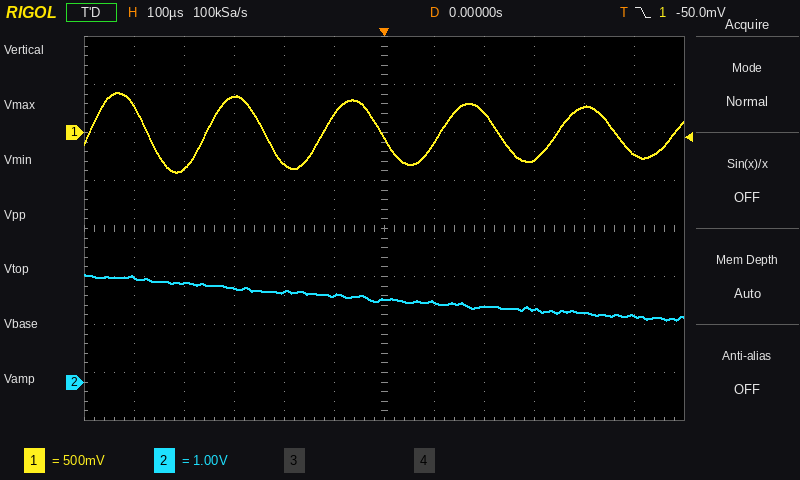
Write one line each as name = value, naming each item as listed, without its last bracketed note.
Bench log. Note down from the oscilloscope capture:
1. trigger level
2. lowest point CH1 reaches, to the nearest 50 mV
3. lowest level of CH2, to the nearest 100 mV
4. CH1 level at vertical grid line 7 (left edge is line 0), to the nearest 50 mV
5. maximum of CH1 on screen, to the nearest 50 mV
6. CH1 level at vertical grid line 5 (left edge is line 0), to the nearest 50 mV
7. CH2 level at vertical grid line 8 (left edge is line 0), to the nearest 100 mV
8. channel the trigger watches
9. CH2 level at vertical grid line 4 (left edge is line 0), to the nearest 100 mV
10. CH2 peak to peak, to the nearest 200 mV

trigger level = -50.0 mV
lowest point CH1 reaches, to the nearest 50 mV = -400 mV
lowest level of CH2, to the nearest 100 mV = 1.3 V
CH1 level at vertical grid line 7 (left edge is line 0), to the nearest 50 mV = -100 mV
maximum of CH1 on screen, to the nearest 50 mV = 400 mV
CH1 level at vertical grid line 5 (left edge is line 0), to the nearest 50 mV = 200 mV
CH2 level at vertical grid line 8 (left edge is line 0), to the nearest 100 mV = 1.6 V
channel the trigger watches = CH1
CH2 level at vertical grid line 4 (left edge is line 0), to the nearest 100 mV = 1.9 V
CH2 peak to peak, to the nearest 200 mV = 1.0 V
